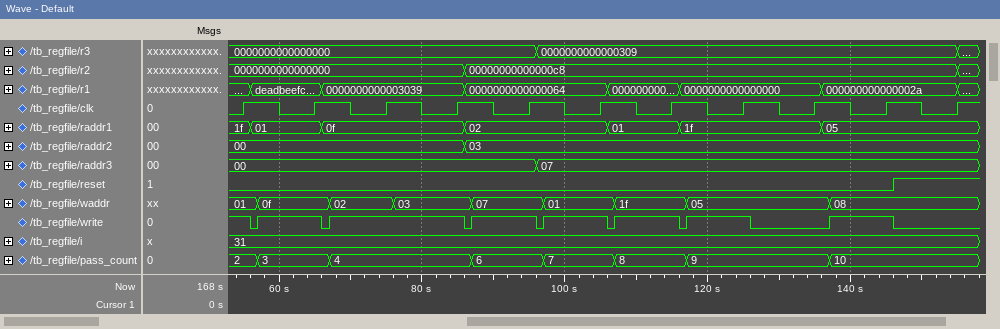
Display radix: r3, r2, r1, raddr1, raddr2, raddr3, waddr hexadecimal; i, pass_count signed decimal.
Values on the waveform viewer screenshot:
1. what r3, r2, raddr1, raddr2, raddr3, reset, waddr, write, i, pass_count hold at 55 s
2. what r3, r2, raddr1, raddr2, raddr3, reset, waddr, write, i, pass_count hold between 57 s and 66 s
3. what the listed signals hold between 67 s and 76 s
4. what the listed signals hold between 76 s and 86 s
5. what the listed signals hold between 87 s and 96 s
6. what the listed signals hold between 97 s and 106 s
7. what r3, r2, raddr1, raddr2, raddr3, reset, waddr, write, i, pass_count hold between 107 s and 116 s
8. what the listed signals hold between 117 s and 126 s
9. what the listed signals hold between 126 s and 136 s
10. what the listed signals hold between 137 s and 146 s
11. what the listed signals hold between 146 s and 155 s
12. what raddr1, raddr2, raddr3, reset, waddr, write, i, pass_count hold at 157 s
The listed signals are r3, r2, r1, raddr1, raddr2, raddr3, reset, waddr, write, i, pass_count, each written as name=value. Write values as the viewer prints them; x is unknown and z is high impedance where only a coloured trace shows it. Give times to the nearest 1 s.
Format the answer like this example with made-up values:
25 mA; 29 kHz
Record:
r3=0000000000000000, r2=0000000000000000, raddr1=1f, raddr2=00, raddr3=00, reset=0, waddr=01, write=1, i=31, pass_count=2; r3=0000000000000000, r2=0000000000000000, raddr1=01, raddr2=00, raddr3=00, reset=0, waddr=0f, write=1, i=31, pass_count=3; r3=0000000000000000, r2=0000000000000000, r1=0000000000003039, raddr1=0f, raddr2=00, raddr3=00, reset=0, waddr=02, write=1, i=31, pass_count=4; r3=0000000000000000, r2=0000000000000000, r1=0000000000003039, raddr1=0f, raddr2=00, raddr3=00, reset=0, waddr=03, write=1, i=31, pass_count=4; r3=0000000000000000, r2=00000000000000c8, r1=0000000000000064, raddr1=02, raddr2=03, raddr3=00, reset=0, waddr=07, write=1, i=31, pass_count=6; r3=0000000000000309, r2=00000000000000c8, r1=0000000000000064, raddr1=02, raddr2=03, raddr3=07, reset=0, waddr=01, write=1, i=31, pass_count=7; r3=0000000000000309, r2=00000000000000c8, raddr1=01, raddr2=03, raddr3=07, reset=0, waddr=1f, write=1, i=31, pass_count=8; r3=0000000000000309, r2=00000000000000c8, r1=0000000000000000, raddr1=1f, raddr2=03, raddr3=07, reset=0, waddr=05, write=1, i=31, pass_count=9; r3=0000000000000309, r2=00000000000000c8, r1=0000000000000000, raddr1=1f, raddr2=03, raddr3=07, reset=0, waddr=05, write=0, i=31, pass_count=9; r3=0000000000000309, r2=00000000000000c8, r1=000000000000002a, raddr1=05, raddr2=03, raddr3=07, reset=0, waddr=08, write=1, i=31, pass_count=10; r3=0000000000000309, r2=00000000000000c8, r1=000000000000002a, raddr1=05, raddr2=03, raddr3=07, reset=1, waddr=08, write=0, i=31, pass_count=10; raddr1=05, raddr2=03, raddr3=07, reset=1, waddr=08, write=0, i=31, pass_count=10
